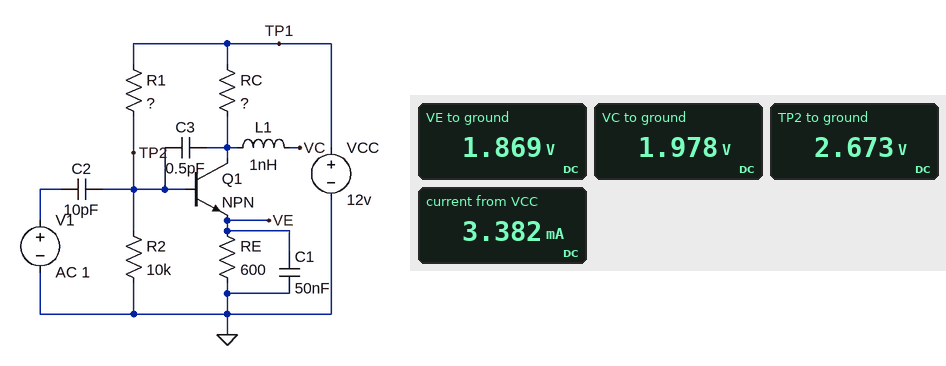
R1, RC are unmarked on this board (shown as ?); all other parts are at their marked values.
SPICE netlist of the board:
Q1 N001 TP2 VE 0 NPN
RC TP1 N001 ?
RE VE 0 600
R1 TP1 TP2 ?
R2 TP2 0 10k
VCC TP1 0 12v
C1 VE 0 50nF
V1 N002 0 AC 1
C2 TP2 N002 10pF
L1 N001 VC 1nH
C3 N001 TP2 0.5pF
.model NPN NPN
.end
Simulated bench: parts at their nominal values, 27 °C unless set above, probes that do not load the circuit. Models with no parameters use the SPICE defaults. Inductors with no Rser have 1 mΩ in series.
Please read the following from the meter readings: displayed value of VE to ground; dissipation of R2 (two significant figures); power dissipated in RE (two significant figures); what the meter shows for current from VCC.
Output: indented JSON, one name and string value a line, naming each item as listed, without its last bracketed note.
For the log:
{
  "displayed value of VE to ground": "1.869 V",
  "dissipation of R2": "710 µW",
  "power dissipated in RE": "5.8 mW",
  "what the meter shows for current from VCC": "3.382 mA"
}
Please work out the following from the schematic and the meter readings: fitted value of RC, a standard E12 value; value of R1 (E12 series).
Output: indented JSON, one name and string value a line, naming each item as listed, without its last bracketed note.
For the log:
{
  "fitted value of RC, a standard E12 value": "3.3 kΩ",
  "value of R1": "27 kΩ"
}
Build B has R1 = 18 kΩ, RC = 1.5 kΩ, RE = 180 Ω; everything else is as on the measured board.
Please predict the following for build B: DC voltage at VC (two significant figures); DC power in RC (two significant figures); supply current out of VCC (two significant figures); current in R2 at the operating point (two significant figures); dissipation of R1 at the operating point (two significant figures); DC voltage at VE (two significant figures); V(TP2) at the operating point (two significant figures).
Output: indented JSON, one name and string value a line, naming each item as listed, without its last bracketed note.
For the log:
{
  "DC voltage at VC": "1.4 V",
  "DC power in RC": "75 mW",
  "supply current out of VCC": "7.6 mA",
  "current in R2 at the operating point": "220 µA",
  "dissipation of R1 at the operating point": "5.4 mW",
  "DC voltage at VE": "1.3 V",
  "V(TP2) at the operating point": "2.2 V"
}
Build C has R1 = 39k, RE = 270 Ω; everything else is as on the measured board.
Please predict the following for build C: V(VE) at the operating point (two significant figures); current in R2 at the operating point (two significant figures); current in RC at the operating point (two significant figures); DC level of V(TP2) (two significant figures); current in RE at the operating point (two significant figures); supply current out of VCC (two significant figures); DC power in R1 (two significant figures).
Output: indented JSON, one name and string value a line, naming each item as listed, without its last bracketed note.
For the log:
{
  "V(VE) at the operating point": "920 mV",
  "current in R2 at the operating point": "170 µA",
  "current in RC at the operating point": "3.3 mA",
  "DC level of V(TP2)": "1.7 V",
  "current in RE at the operating point": "3.4 mA",
  "supply current out of VCC": "3.6 mA",
  "DC power in R1": "2.7 mW"
}
